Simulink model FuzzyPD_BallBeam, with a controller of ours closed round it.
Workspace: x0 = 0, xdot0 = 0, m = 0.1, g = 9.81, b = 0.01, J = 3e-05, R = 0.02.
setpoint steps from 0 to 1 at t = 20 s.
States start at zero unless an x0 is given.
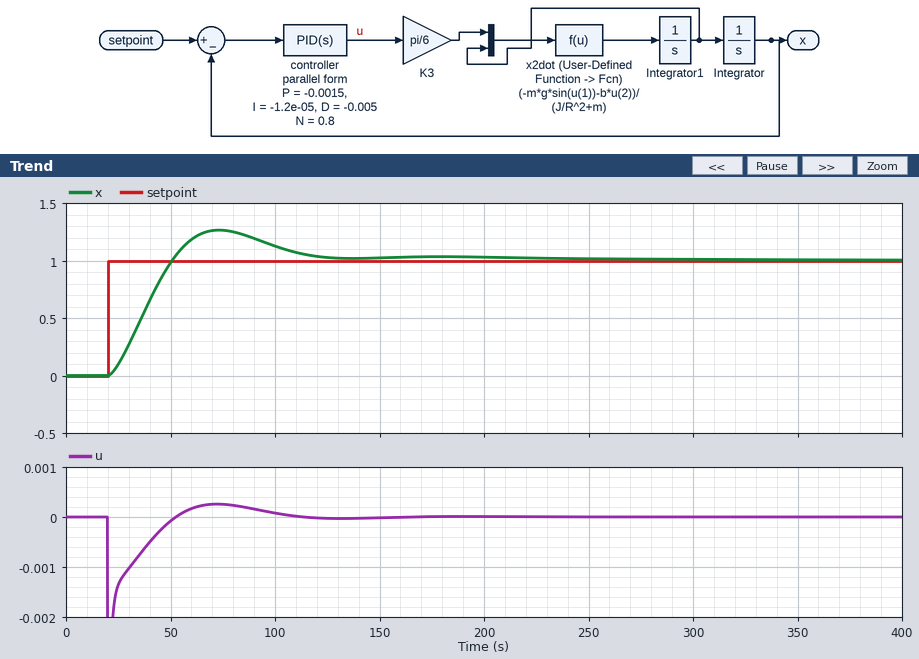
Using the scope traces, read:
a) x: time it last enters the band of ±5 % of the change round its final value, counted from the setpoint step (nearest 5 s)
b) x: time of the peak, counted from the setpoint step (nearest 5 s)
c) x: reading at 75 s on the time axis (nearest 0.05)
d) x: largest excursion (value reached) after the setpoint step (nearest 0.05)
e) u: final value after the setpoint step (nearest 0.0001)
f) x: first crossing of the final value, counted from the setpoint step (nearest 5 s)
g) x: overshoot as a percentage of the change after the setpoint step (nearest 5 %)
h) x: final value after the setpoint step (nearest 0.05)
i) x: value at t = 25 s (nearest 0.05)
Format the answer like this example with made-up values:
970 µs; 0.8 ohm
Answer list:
95 s; 55 s; 1.25; 1.25; 0.0000; 30 s; 25 %; 1.00; 0.10
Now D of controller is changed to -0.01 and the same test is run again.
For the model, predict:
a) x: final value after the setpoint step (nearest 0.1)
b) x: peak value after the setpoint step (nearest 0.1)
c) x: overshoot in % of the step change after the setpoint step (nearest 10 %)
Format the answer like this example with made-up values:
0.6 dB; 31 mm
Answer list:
1.0; 1.2; 20 %
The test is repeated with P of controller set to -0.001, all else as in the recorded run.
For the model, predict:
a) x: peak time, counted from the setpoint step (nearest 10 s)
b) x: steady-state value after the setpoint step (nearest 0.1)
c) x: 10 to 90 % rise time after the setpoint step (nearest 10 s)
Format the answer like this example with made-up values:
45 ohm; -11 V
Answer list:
70 s; 1.0; 30 s
